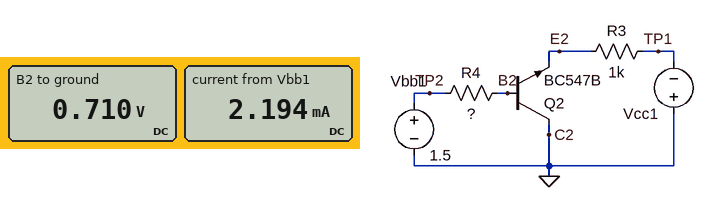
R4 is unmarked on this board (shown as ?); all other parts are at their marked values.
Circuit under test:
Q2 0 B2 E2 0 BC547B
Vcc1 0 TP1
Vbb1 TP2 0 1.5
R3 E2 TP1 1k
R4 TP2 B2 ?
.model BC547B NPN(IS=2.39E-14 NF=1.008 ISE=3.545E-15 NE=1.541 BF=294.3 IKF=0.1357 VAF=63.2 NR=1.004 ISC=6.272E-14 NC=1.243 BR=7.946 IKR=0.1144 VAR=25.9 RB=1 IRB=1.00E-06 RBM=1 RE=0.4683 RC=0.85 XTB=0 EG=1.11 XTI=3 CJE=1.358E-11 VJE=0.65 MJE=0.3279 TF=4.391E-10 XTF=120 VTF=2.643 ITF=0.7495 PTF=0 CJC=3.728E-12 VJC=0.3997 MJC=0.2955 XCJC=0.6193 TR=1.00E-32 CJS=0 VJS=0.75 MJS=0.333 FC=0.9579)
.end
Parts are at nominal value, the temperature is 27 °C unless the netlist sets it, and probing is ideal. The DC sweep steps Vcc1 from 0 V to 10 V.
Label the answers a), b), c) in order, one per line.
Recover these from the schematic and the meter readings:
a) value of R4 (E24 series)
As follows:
a) 360 Ω
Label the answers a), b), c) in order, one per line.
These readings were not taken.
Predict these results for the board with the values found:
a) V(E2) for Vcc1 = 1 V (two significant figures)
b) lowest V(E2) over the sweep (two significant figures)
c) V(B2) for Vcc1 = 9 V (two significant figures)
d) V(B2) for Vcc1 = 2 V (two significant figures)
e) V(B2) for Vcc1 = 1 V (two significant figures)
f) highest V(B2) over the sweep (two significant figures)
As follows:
a) -4.2 mV
b) -30 mV
c) 700 mV
d) 710 mV
e) 710 mV
f) 710 mV
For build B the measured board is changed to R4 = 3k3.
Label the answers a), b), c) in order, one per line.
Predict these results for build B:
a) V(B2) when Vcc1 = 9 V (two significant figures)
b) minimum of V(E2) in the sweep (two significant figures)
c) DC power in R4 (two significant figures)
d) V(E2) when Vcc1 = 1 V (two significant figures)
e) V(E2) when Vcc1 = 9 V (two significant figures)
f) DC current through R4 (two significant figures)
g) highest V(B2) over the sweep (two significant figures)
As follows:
a) 640 mV
b) -72 mV
c) 220 µW
d) -16 mV
e) -67 mV
f) 260 µA
g) 650 mV
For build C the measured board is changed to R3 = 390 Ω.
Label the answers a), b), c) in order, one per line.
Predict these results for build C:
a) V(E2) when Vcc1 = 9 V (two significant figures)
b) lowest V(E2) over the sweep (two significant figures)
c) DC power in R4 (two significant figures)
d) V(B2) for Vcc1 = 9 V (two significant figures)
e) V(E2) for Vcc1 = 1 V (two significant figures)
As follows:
a) -61 mV
b) -67 mV
c) 1.7 mW
d) 690 mV
e) -9.2 mV
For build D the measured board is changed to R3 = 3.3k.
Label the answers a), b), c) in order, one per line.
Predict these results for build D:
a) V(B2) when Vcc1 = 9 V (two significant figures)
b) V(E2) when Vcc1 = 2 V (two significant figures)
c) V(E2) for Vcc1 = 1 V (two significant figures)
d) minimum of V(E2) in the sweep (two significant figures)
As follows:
a) 710 mV
b) -2.9 mV
c) -1.9 mV
d) -11 mV
